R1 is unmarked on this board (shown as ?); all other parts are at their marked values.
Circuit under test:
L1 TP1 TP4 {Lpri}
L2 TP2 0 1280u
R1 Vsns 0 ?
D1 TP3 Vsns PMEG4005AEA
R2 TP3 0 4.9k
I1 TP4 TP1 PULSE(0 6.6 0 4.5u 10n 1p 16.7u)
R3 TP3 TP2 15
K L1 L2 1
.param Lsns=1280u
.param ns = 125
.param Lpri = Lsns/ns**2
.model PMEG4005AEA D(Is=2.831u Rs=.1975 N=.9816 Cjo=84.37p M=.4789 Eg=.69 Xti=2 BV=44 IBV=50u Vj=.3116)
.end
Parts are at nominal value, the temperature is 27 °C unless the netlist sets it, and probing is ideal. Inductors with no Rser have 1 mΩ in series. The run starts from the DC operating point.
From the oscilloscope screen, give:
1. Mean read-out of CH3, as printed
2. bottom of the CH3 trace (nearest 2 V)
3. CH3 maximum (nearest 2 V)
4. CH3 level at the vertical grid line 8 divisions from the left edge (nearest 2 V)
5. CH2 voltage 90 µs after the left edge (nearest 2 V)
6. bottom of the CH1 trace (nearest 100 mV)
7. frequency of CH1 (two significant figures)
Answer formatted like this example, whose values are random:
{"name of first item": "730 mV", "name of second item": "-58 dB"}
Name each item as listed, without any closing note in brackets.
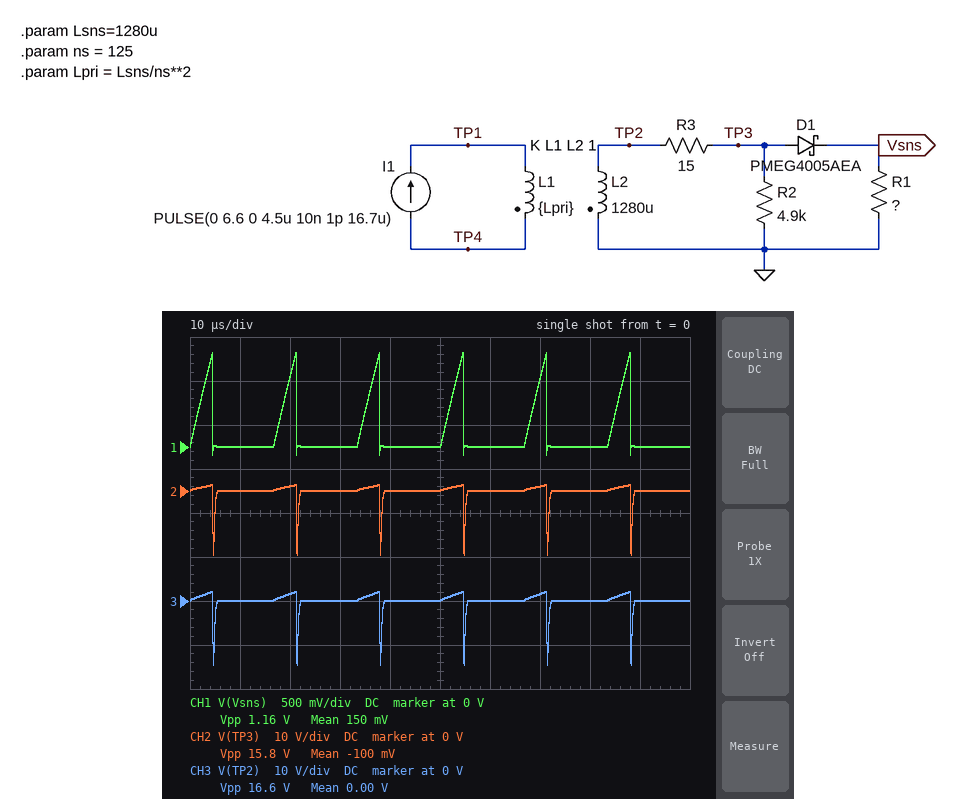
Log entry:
{"Mean read-out of CH3, as printed": "0.00 V", "bottom of the CH3 trace": "-14 V", "CH3 maximum": "2 V", "CH3 level at the vertical grid line 8 divisions from the left edge": "0 V", "CH2 voltage 90 µs after the left edge": "0 V", "bottom of the CH1 trace": "-100 mV", "frequency of CH1": "60 kHz"}
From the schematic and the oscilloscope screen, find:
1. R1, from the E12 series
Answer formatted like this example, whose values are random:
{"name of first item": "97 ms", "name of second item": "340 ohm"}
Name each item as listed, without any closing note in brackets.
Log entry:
{"R1, from the E12 series": "22 Ω"}
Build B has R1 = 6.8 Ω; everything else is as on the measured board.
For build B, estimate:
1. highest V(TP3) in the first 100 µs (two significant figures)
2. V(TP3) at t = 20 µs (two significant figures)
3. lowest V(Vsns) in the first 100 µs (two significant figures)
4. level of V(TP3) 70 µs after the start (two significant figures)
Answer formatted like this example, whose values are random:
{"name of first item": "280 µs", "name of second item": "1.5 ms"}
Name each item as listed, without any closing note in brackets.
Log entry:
{"highest V(TP3) in the first 100 µs": "600 mV", "V(TP3) at t = 20 µs": "500 mV", "lowest V(Vsns) in the first 100 µs": "-19 mV", "level of V(TP3) 70 µs after the start": "490 mV"}
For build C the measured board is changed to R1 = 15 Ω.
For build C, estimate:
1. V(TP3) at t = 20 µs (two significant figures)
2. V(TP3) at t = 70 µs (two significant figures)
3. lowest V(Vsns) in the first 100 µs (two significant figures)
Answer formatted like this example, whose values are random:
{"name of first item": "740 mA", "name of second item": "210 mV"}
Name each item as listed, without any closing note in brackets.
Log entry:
{"V(TP3) at t = 20 µs": "800 mV", "V(TP3) at t = 70 µs": "780 mV", "lowest V(Vsns) in the first 100 µs": "-52 mV"}
